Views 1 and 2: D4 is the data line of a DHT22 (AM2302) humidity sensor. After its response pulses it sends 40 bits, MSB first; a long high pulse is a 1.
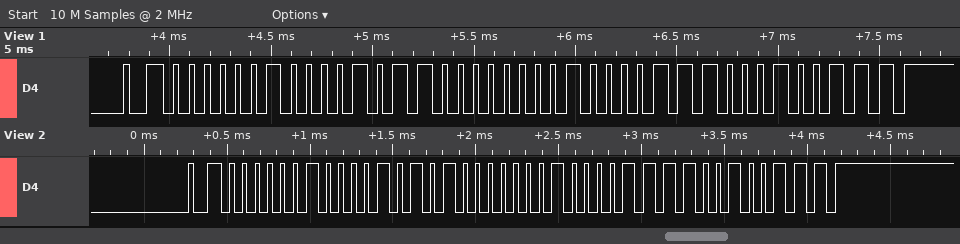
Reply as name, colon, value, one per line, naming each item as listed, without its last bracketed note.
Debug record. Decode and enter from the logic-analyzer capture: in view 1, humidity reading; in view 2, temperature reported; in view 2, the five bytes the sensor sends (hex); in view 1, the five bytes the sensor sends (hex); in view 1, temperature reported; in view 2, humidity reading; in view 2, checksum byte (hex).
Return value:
in view 1, humidity reading: 53.4 %
in view 2, temperature reported: 27.1 °C
in view 2, the five bytes the sensor sends: 02 15 01 0F 27
in view 1, the five bytes the sensor sends: 02 16 01 0E 27
in view 1, temperature reported: 27.0 °C
in view 2, humidity reading: 53.3 %
in view 2, checksum byte: 0x27
